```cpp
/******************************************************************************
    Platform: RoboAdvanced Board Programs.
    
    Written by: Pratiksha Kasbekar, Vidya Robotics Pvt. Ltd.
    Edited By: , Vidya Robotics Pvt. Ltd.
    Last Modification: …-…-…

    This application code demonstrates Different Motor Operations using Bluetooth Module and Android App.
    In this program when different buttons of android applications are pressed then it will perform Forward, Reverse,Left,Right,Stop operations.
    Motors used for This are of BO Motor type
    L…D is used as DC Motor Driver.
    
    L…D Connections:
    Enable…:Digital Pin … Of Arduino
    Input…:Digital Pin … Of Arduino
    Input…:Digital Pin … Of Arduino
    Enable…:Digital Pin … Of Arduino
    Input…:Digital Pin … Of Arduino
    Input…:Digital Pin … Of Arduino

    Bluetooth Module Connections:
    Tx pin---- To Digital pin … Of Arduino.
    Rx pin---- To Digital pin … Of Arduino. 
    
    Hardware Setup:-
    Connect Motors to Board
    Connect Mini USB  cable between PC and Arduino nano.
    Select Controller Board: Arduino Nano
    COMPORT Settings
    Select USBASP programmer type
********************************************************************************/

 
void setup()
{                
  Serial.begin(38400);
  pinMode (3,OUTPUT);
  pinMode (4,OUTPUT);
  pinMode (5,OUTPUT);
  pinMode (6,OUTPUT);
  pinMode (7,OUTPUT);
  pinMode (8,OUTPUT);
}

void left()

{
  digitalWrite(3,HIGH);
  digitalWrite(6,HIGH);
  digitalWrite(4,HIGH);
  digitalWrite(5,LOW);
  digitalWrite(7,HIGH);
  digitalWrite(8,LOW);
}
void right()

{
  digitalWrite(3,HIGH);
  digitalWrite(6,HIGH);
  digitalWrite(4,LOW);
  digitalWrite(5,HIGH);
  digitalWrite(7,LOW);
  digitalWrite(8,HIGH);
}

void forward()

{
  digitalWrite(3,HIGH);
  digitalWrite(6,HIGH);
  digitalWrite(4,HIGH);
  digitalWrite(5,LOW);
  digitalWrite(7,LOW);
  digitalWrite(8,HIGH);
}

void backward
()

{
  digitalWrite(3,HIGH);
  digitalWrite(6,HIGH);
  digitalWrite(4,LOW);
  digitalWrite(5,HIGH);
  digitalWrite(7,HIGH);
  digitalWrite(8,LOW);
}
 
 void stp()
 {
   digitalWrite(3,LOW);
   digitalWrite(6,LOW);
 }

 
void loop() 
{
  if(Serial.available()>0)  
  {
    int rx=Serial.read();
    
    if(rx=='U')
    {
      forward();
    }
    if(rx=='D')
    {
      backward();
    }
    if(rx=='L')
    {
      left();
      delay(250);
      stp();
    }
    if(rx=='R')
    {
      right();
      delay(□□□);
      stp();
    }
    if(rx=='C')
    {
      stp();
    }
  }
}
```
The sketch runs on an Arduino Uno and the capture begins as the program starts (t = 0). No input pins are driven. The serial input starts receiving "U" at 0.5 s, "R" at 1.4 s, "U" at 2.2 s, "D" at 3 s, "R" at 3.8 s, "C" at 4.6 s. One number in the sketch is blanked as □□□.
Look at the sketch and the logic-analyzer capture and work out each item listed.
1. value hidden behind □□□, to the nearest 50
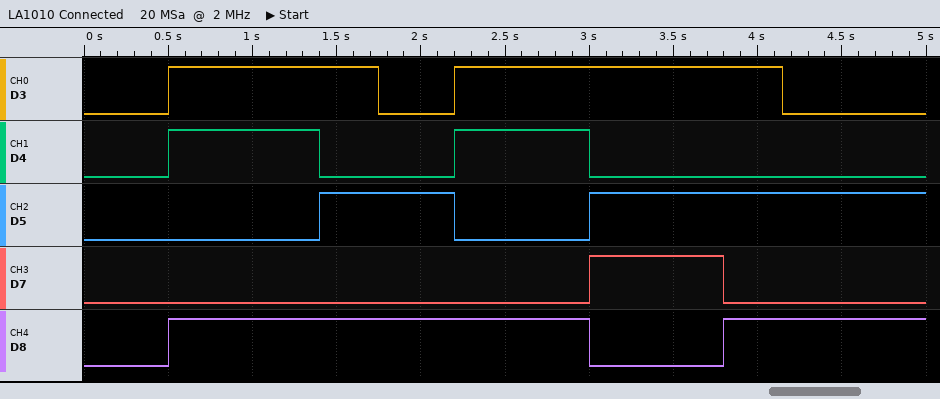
350
